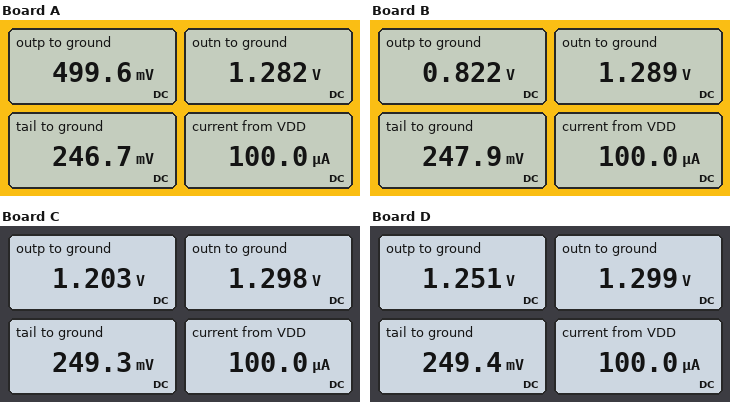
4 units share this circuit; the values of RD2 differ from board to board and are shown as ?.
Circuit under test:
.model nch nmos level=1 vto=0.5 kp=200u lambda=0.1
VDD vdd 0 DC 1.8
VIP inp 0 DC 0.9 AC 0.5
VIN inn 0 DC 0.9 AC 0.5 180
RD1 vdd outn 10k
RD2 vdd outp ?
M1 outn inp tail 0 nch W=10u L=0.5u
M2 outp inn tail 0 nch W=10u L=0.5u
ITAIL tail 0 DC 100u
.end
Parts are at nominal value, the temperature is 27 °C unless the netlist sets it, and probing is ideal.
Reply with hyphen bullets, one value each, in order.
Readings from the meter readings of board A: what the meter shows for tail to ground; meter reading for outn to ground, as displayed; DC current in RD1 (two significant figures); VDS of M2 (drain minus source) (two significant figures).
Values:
- 246.7 mV
- 1.282 V
- 52 µA
- 250 mV
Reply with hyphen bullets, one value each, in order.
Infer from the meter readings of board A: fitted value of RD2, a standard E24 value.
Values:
- 27 kΩ
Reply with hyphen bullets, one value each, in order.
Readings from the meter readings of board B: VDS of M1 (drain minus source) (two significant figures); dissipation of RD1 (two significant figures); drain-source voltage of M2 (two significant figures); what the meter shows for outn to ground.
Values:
- 1.0 V
- 26 µW
- 570 mV
- 1.289 V
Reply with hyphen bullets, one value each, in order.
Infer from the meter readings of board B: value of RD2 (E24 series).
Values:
- 20 kΩ
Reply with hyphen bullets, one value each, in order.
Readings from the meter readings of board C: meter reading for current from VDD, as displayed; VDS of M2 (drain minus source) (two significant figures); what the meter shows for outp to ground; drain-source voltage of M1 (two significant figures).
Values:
- 100.0 µA
- 950 mV
- 1.203 V
- 1.0 V
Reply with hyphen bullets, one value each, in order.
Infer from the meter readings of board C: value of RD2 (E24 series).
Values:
- 12 kΩ
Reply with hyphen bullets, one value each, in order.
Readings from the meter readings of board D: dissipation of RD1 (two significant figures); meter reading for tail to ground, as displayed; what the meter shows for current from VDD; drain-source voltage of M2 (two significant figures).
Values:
- 25 µW
- 249.4 mV
- 100.0 µA
- 1.0 V
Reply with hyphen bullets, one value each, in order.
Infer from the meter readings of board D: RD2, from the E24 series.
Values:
- 11 kΩ
